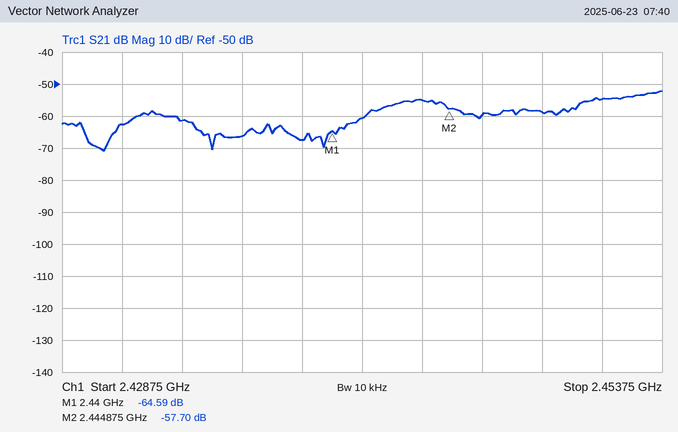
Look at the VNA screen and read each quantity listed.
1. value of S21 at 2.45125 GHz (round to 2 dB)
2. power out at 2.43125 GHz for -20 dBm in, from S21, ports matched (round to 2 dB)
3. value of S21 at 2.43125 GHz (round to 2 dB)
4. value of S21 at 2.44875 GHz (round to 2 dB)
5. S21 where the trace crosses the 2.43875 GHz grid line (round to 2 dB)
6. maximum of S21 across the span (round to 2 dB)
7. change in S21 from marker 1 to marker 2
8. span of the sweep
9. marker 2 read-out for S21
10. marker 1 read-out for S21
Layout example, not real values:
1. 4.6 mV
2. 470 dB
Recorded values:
1. -54 dB
2. -82 dBm
3. -62 dB
4. -58 dB
5. -68 dB
6. -52 dB
7. 6.89 dB
8. 25 MHz
9. -57.70 dB
10. -64.59 dB
